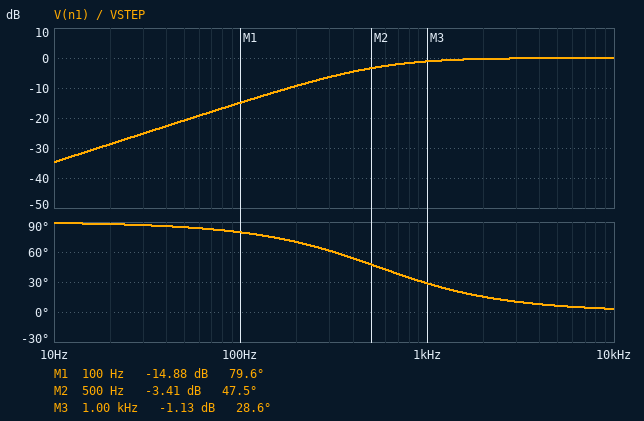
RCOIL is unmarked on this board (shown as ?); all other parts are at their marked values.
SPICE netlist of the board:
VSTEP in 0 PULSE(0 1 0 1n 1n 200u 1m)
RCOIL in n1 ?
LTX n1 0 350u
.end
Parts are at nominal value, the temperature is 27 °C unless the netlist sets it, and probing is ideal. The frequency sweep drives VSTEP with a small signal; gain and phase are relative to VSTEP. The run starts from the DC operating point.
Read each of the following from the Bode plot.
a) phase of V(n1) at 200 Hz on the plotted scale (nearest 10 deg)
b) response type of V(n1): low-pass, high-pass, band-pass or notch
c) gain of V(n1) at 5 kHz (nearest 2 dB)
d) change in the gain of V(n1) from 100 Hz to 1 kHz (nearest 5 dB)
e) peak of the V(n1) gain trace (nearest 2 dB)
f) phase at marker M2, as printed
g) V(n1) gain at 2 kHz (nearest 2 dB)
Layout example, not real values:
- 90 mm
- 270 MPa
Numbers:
- 70 deg
- high-pass
- 0 dB
- 15 dB
- 0 dB
- 47.5 deg
- 0 dB
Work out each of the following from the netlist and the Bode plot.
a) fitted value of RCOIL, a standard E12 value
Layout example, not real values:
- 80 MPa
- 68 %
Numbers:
- 1.2 Ω
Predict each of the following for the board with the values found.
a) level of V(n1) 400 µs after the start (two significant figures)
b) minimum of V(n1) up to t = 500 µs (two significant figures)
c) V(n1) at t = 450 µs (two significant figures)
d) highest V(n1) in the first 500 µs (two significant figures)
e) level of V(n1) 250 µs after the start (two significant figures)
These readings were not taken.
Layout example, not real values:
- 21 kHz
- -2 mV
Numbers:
- -250 mV
- -500 mV
- -210 mV
- 1.0 V
- -420 mV
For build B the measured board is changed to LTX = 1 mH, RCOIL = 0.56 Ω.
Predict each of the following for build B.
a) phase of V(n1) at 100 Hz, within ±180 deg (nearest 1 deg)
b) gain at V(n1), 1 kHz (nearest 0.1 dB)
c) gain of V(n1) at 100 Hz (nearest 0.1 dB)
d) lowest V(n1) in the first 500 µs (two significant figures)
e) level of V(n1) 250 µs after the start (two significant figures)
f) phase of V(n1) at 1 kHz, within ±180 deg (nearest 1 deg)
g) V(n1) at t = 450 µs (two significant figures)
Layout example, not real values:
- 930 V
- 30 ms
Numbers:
- 42 deg
- 0 dB
- -2.5 dB
- -110 mV
- -100 mV
- 5 deg
- -92 mV
